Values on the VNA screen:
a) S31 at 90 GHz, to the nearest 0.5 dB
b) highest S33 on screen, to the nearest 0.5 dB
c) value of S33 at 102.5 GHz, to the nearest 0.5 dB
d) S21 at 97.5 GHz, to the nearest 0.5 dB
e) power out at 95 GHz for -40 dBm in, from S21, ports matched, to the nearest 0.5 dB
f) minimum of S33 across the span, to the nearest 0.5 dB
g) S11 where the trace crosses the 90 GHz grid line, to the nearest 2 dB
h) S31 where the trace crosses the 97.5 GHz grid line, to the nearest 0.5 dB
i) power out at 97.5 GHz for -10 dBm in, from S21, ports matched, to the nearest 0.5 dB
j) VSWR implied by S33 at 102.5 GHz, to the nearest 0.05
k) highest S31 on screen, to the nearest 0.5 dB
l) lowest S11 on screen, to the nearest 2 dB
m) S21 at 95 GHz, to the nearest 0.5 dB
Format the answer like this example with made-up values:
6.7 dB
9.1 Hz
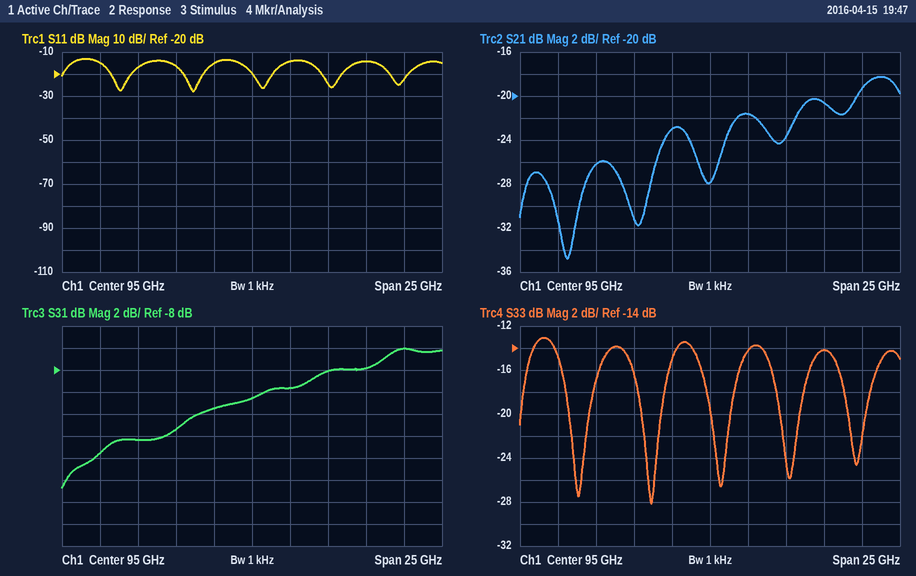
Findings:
-13.5 dB
-13.0 dB
-14.0 dB
-21.5 dB
-68.0 dBm
-28.0 dB
-16 dB
-9.5 dB
-31.5 dBm
1.50
-6.0 dB
-28 dB
-28.0 dB
